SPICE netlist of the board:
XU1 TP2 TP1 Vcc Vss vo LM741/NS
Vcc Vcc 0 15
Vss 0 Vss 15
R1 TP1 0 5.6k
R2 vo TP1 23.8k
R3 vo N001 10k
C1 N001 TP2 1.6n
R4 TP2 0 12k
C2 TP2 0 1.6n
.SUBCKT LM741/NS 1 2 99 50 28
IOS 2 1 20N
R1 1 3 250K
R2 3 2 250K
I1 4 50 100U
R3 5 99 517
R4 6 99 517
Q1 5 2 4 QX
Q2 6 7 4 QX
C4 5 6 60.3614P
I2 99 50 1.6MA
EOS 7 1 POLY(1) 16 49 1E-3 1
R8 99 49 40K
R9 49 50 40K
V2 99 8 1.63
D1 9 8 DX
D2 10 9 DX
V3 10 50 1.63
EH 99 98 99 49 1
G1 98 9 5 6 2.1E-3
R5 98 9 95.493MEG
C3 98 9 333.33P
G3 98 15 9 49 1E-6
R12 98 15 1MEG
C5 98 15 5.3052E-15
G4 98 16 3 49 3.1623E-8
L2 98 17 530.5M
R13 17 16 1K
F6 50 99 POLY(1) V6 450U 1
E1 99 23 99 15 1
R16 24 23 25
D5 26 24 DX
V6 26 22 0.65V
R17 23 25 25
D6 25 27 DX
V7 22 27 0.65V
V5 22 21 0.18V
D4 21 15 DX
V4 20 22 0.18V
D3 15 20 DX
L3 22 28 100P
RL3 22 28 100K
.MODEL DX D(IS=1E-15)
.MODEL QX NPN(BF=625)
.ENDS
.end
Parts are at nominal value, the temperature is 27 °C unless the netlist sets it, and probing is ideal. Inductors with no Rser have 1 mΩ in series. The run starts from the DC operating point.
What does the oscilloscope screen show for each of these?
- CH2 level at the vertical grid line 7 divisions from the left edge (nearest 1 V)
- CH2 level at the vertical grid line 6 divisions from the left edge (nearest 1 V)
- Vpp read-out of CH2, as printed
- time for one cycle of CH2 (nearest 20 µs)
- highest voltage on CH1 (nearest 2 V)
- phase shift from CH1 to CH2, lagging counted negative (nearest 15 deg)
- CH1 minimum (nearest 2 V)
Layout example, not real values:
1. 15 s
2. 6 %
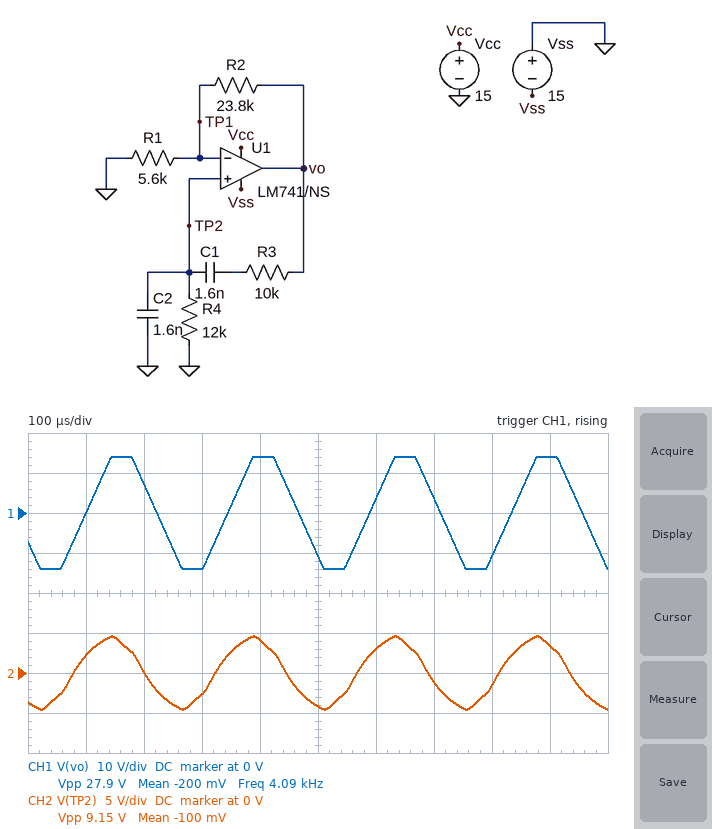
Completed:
1. -1 V
2. 3 V
3. 9.15 V
4. 240 µs
5. 14 V
6. 30 deg
7. -14 V
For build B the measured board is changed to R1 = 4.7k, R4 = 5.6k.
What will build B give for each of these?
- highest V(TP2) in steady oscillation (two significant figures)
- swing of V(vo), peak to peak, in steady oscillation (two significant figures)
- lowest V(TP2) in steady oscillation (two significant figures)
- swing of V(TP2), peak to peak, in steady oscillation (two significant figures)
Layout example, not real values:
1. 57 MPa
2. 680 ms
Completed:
1. 2.6 V
2. 28 V
3. -2.6 V
4. 5.2 V
